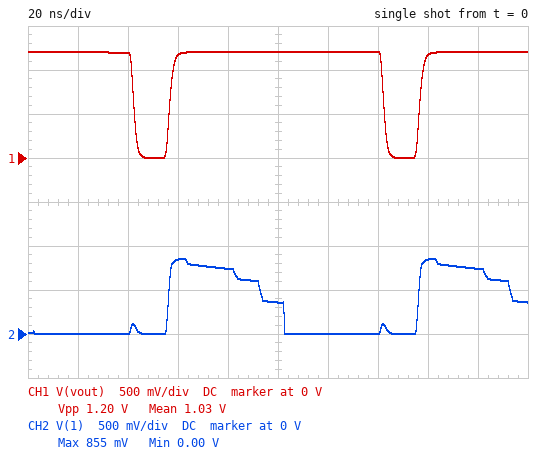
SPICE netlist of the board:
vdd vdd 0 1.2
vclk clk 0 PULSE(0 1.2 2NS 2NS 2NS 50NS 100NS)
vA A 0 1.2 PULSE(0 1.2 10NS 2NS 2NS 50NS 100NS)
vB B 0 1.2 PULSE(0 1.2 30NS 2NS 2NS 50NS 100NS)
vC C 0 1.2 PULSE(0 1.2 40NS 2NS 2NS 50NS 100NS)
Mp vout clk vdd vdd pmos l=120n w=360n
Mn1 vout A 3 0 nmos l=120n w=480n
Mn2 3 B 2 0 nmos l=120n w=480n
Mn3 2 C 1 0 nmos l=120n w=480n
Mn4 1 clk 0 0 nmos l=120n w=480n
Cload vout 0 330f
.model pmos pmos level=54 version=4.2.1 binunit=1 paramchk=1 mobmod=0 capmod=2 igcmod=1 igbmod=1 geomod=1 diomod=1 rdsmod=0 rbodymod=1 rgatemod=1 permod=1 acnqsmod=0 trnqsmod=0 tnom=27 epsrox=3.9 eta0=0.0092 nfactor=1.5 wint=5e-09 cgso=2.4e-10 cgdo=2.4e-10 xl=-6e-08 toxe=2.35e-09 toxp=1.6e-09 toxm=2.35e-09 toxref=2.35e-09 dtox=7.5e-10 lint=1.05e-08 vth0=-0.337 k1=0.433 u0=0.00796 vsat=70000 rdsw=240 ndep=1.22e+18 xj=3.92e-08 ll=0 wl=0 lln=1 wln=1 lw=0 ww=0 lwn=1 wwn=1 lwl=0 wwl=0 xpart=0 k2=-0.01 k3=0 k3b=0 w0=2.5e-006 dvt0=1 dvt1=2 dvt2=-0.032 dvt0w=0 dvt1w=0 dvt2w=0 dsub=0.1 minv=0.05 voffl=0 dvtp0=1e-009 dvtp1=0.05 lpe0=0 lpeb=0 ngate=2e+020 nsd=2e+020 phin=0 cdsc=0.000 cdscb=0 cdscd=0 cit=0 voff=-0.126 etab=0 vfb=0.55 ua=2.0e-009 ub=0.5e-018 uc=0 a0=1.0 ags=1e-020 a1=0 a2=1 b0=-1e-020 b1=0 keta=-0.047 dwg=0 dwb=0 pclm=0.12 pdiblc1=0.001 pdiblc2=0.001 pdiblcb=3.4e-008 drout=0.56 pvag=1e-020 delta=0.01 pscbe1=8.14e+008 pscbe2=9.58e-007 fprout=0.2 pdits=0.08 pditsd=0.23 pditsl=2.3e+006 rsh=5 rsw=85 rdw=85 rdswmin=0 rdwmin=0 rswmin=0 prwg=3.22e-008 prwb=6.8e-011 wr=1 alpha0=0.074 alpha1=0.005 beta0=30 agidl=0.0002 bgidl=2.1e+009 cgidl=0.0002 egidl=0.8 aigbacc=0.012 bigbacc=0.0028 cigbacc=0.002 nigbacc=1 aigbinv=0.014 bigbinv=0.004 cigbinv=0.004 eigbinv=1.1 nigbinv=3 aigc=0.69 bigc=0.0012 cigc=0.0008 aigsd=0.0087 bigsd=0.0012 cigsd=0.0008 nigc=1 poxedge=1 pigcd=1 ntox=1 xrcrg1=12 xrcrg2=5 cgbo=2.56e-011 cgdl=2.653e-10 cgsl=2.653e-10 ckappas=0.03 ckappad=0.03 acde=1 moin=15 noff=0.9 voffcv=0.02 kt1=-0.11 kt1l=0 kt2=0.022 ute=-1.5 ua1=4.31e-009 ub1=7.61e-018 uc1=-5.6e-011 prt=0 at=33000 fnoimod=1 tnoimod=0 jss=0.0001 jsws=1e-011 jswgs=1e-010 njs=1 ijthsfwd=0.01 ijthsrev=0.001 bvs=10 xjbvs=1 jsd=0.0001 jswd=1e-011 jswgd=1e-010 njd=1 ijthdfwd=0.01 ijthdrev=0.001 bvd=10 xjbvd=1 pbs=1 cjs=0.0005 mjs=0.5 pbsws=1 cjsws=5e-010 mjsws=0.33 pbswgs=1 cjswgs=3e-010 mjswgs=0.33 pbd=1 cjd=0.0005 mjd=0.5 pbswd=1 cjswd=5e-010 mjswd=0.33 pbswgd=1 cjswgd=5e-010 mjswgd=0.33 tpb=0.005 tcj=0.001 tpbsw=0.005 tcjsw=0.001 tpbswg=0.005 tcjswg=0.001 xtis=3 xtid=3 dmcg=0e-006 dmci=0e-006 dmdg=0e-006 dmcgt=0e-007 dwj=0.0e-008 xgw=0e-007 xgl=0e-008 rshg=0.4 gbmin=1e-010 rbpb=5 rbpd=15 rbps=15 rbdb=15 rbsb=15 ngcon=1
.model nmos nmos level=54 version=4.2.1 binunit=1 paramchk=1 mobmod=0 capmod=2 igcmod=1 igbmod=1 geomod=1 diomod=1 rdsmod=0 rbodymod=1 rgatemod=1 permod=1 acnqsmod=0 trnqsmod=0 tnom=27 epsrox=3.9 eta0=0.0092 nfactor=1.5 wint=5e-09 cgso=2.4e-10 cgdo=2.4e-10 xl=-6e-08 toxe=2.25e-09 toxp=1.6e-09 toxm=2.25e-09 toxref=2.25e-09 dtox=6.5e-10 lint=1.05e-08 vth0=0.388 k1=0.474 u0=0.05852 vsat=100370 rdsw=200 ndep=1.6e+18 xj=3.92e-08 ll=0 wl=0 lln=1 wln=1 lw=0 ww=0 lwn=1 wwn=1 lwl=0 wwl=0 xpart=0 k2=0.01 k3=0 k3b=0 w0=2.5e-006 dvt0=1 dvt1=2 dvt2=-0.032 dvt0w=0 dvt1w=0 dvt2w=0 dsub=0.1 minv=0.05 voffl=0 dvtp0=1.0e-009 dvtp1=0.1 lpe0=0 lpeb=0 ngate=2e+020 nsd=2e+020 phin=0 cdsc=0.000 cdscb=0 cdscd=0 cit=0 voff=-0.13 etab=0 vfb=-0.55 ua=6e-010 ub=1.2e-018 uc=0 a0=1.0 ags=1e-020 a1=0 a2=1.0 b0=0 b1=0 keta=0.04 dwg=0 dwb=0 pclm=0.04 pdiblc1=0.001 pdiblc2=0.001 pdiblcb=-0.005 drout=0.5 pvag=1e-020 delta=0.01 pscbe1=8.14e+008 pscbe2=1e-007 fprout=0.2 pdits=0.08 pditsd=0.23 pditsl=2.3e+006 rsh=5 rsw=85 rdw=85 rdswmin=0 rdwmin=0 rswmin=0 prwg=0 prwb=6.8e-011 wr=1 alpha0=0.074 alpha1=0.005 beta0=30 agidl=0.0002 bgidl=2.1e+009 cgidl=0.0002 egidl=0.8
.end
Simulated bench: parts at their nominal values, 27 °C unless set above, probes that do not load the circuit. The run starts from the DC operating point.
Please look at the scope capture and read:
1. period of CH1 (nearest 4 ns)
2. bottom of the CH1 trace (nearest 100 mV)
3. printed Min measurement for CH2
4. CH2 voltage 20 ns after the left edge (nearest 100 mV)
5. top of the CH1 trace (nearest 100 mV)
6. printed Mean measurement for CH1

100 ns
0 V
0.00 V
0 V
1.2 V
1.03 V
